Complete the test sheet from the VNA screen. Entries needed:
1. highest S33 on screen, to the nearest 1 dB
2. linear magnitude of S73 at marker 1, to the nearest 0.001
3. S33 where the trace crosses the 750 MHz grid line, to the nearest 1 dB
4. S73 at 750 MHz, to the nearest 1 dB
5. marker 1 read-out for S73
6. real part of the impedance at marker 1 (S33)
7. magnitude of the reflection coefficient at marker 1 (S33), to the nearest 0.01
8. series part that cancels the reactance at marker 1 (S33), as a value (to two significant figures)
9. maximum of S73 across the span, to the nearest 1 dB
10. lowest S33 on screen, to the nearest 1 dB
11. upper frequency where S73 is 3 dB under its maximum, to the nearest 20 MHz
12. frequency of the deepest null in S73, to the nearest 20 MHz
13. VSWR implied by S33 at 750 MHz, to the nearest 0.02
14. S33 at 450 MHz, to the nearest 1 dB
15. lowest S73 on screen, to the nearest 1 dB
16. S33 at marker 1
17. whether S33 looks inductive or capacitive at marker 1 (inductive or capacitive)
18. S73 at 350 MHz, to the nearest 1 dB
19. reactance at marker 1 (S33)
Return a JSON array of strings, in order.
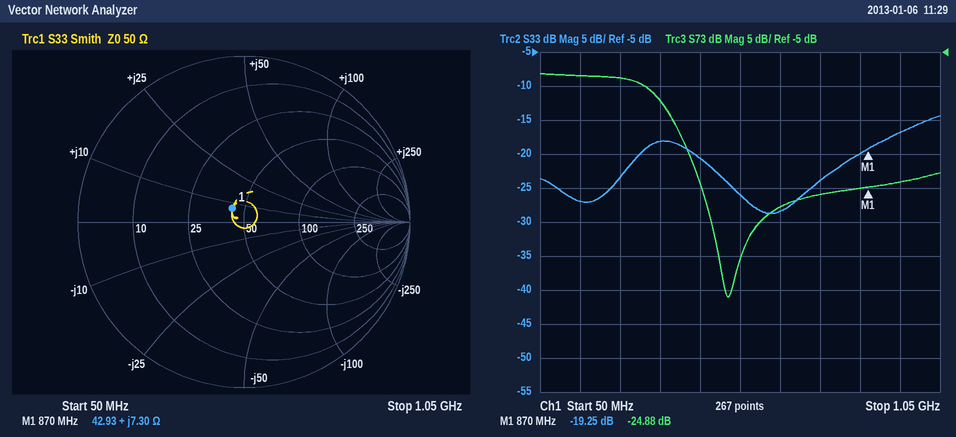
["-14 dB", "0.057", "-24 dB", "-26 dB", "-24.88 dB", "42.93 Ω", "0.11", "25 pF", "-8 dB", "-29 dB", "340 MHz", "520 MHz", "1.14", "-21 dB", "-41 dB", "-19.25 dB", "inductive", "-12 dB", "+7.30 Ω"]
